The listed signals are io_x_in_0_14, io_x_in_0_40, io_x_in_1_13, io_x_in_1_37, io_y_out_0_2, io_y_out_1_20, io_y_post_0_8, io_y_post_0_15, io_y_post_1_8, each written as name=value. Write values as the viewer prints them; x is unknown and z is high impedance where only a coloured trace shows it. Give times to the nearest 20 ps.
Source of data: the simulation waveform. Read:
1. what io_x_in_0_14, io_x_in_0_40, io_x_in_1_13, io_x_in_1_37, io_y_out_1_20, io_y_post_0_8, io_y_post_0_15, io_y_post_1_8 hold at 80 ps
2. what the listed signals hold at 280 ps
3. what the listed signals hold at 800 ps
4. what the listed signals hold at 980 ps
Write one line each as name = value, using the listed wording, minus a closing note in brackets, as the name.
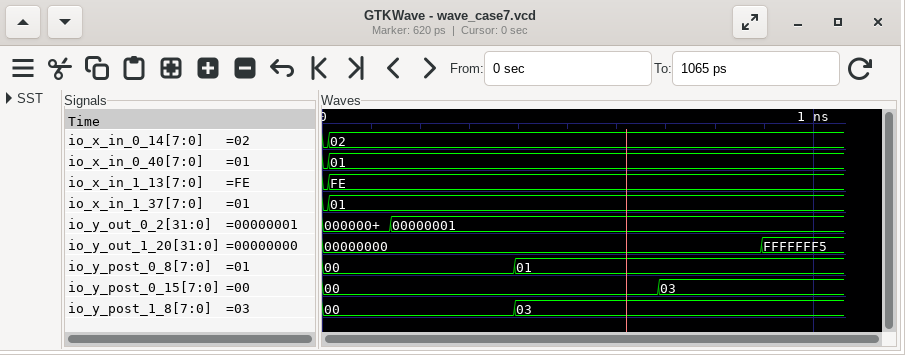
what io_x_in_0_14, io_x_in_0_40, io_x_in_1_13, io_x_in_1_37, io_y_out_1_20, io_y_post_0_8, io_y_post_0_15, io_y_post_1_8 hold at 80 ps = io_x_in_0_14=02, io_x_in_0_40=01, io_x_in_1_13=FE, io_x_in_1_37=01, io_y_out_1_20=00000000, io_y_post_0_8=00, io_y_post_0_15=00, io_y_post_1_8=00
what the listed signals hold at 280 ps = io_x_in_0_14=02, io_x_in_0_40=01, io_x_in_1_13=FE, io_x_in_1_37=01, io_y_out_0_2=00000001, io_y_out_1_20=00000000, io_y_post_0_8=00, io_y_post_0_15=00, io_y_post_1_8=00
what the listed signals hold at 800 ps = io_x_in_0_14=02, io_x_in_0_40=01, io_x_in_1_13=FE, io_x_in_1_37=01, io_y_out_0_2=00000001, io_y_out_1_20=00000000, io_y_post_0_8=01, io_y_post_0_15=03, io_y_post_1_8=03
what the listed signals hold at 980 ps = io_x_in_0_14=02, io_x_in_0_40=01, io_x_in_1_13=FE, io_x_in_1_37=01, io_y_out_0_2=00000001, io_y_out_1_20=FFFFFFF5, io_y_post_0_8=01, io_y_post_0_15=03, io_y_post_1_8=03
